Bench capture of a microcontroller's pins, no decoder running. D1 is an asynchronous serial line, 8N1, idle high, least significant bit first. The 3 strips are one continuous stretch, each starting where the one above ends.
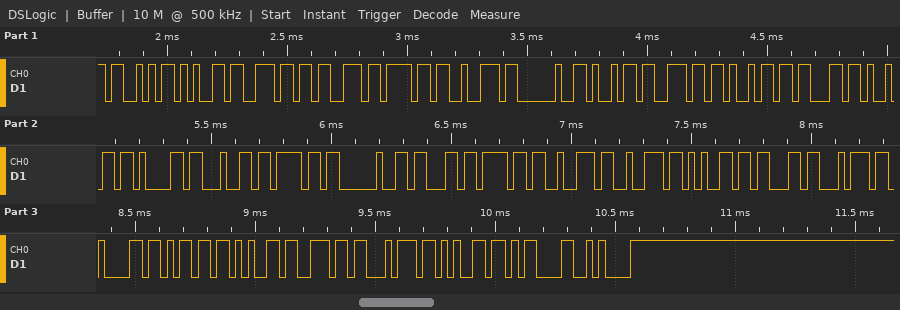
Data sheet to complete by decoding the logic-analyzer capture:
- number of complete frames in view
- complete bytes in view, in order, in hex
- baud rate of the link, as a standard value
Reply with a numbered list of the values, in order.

1. 31
2. 53 65 6E 73 6F 72 20 69 6E 69 63 69 61 64 6F 20 63 6F 72 72 65 63 74 61 6D 65 6E 74 65 0D 0A
3. 38400 baud
